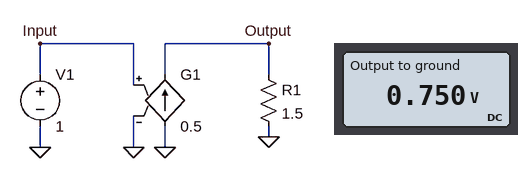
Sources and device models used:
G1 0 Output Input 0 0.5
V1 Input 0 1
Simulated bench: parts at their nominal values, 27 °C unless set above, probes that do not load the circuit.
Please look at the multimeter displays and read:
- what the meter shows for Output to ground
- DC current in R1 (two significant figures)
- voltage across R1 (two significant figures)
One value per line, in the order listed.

0.750 V
500 mA
750 mV
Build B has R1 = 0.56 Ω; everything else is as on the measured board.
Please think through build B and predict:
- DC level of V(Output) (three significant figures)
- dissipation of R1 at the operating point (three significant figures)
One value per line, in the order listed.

280 mV
140 mW
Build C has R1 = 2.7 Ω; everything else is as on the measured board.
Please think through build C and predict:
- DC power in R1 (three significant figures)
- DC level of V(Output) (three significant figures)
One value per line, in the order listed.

675 mW
1.35 V
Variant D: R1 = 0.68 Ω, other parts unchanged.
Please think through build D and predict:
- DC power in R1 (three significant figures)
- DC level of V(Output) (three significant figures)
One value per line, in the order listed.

170 mW
340 mV
